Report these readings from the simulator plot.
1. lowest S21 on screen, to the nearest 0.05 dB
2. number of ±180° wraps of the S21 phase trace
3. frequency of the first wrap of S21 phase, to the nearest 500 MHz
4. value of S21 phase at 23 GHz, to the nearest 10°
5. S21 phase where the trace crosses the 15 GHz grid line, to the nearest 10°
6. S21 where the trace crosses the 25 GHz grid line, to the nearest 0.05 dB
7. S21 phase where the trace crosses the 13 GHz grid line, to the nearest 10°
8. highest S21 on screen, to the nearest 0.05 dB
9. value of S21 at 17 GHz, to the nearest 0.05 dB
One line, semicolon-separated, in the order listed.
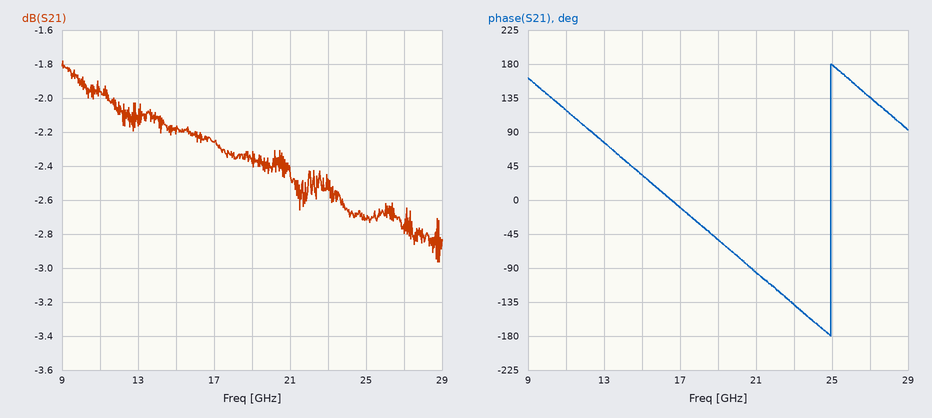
-2.95 dB; 1; 25.0 GHz; -140°; 30°; -2.70 dB; 80°; -1.80 dB; -2.25 dB
